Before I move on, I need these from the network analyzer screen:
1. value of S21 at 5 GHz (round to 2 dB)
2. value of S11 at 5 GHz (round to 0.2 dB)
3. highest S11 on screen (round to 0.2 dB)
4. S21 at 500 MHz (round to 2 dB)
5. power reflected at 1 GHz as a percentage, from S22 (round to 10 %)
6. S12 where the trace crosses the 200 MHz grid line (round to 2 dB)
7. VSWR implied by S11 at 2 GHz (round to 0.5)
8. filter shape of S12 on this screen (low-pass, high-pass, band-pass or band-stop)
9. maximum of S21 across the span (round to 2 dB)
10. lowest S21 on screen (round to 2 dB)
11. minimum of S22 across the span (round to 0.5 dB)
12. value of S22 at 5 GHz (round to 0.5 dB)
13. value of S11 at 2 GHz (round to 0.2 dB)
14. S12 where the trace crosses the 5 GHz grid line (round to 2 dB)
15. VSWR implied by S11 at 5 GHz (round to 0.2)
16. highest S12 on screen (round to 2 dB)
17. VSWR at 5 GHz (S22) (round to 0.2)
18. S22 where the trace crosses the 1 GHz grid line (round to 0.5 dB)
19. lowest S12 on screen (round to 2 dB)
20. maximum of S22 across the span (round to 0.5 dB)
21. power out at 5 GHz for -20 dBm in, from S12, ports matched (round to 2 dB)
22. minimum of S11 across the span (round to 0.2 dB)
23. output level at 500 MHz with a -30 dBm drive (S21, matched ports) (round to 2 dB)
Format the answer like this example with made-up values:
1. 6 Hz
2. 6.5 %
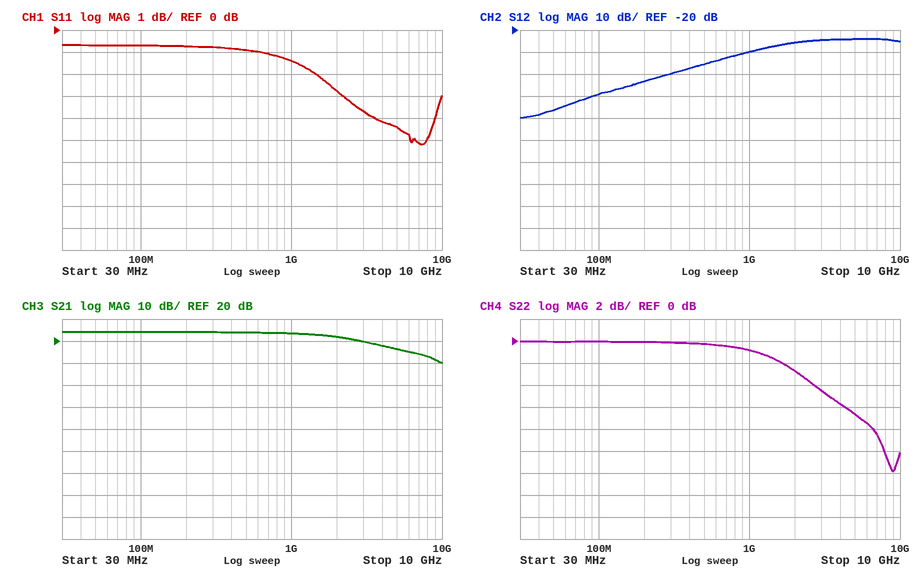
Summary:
1. 16 dB
2. -4.4 dB
3. -0.6 dB
4. 24 dB
5. 80 %
6. -44 dB
7. 6.5
8. high-pass
9. 24 dB
10. 10 dB
11. -12.0 dB
12. -6.5 dB
13. -2.8 dB
14. -24 dB
15. 4.0
16. -24 dB
17. 2.8
18. -1.0 dB
19. -60 dB
20. 0.0 dB
21. -44 dBm
22. -5.2 dB
23. -6 dBm
